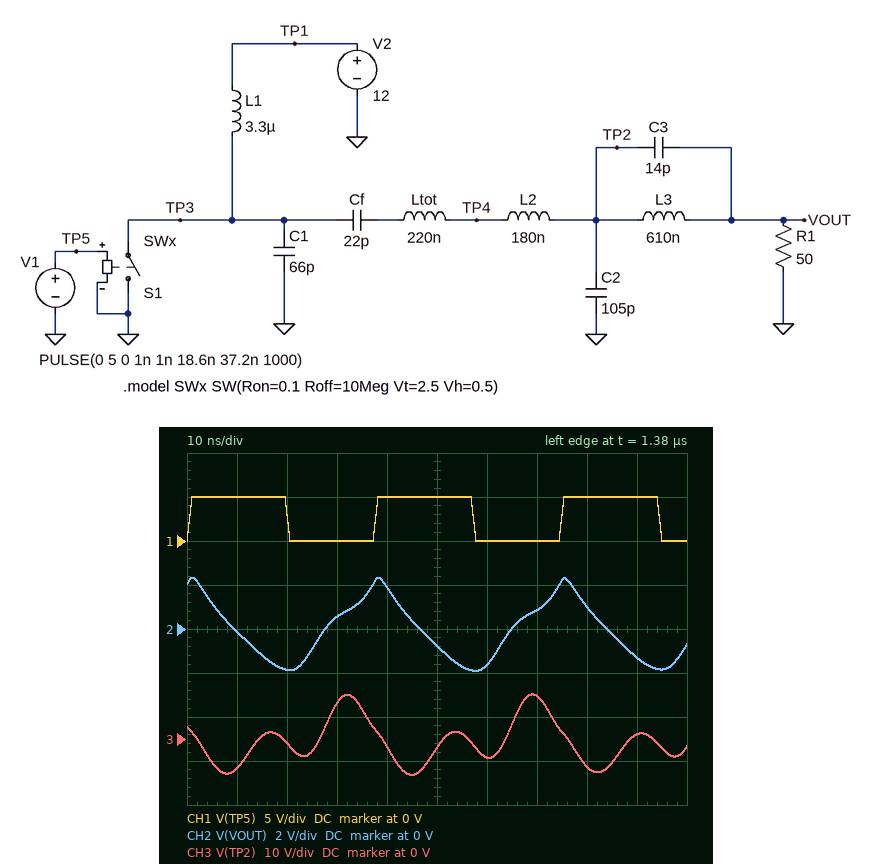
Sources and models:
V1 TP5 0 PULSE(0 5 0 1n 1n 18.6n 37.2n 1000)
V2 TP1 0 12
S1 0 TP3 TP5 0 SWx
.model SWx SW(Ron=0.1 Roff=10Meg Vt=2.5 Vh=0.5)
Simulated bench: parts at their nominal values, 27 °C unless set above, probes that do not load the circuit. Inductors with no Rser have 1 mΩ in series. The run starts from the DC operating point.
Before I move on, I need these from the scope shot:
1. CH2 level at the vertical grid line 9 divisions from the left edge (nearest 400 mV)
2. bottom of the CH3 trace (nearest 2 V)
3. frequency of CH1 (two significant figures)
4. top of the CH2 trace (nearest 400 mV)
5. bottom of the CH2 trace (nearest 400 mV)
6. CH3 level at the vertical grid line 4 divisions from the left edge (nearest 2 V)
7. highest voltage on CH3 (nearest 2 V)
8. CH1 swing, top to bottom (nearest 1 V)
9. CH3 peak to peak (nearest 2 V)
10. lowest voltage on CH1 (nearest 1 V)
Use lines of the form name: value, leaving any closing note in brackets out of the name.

CH2 level at the vertical grid line 9 divisions from the left edge: -1.2 V
bottom of the CH3 trace: -8 V
frequency of CH1: 27 MHz
top of the CH2 trace: 2.4 V
bottom of the CH2 trace: -2.0 V
CH3 level at the vertical grid line 4 divisions from the left edge: -2 V
highest voltage on CH3: 10 V
CH1 swing, top to bottom: 5 V
CH3 peak to peak: 18 V
lowest voltage on CH1: 0 V
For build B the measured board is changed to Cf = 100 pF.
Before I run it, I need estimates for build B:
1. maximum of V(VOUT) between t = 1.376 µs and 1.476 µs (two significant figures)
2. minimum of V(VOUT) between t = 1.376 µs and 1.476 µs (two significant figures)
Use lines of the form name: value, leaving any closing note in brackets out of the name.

maximum of V(VOUT) between t = 1.376 µs and 1.476 µs: 7.7 V
minimum of V(VOUT) between t = 1.376 µs and 1.476 µs: -7.8 V
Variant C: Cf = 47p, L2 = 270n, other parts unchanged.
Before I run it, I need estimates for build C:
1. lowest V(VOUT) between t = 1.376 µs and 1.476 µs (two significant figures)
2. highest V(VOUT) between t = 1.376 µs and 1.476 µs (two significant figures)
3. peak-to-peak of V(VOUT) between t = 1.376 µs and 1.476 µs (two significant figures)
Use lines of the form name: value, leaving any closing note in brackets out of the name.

lowest V(VOUT) between t = 1.376 µs and 1.476 µs: -4.8 V
highest V(VOUT) between t = 1.376 µs and 1.476 µs: 4.9 V
peak-to-peak of V(VOUT) between t = 1.376 µs and 1.476 µs: 9.7 V
